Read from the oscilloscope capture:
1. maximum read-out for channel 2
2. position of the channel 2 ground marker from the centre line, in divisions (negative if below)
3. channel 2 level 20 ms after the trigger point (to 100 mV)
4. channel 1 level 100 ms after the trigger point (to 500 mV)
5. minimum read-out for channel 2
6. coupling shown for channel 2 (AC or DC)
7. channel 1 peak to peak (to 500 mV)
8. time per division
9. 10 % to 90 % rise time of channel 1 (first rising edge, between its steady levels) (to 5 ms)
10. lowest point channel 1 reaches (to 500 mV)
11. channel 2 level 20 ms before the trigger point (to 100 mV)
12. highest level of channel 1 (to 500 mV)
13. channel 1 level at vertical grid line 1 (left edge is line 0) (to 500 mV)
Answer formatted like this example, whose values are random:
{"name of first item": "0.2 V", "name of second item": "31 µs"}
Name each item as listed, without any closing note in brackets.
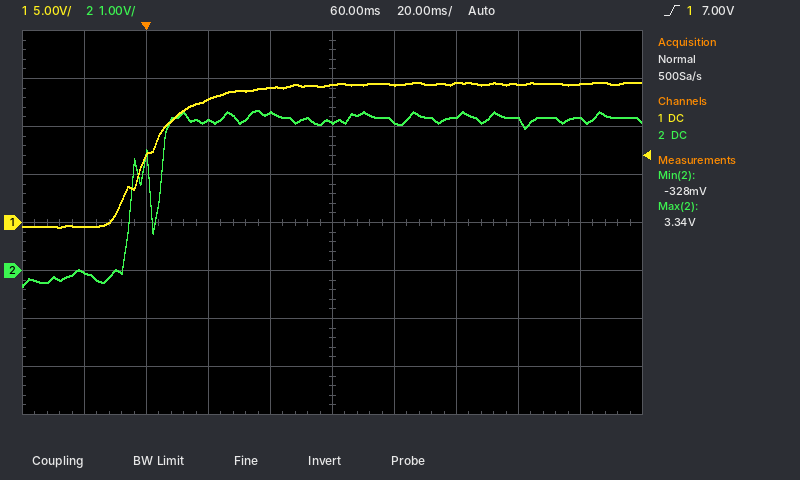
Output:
{"maximum read-out for channel 2": "3.34 V", "position of the channel 2 ground marker from the centre line, in divisions": "-1.0 div", "channel 2 level 20 ms after the trigger point": "3.1 V", "channel 1 level 100 ms after the trigger point": "14.5 V", "minimum read-out for channel 2": "-328 mV", "coupling shown for channel 2": "DC", "channel 1 peak to peak": "15.0 V", "time per division": "20 ms", "10 % to 90 % rise time of channel 1 (first rising edge, between its steady levels)": "30 ms", "lowest point channel 1 reaches": "-500 mV", "channel 2 level 20 ms before the trigger point": "0.0 V", "highest level of channel 1": "14.5 V", "channel 1 level at vertical grid line 1 (left edge is line 0)": "-500 mV"}
